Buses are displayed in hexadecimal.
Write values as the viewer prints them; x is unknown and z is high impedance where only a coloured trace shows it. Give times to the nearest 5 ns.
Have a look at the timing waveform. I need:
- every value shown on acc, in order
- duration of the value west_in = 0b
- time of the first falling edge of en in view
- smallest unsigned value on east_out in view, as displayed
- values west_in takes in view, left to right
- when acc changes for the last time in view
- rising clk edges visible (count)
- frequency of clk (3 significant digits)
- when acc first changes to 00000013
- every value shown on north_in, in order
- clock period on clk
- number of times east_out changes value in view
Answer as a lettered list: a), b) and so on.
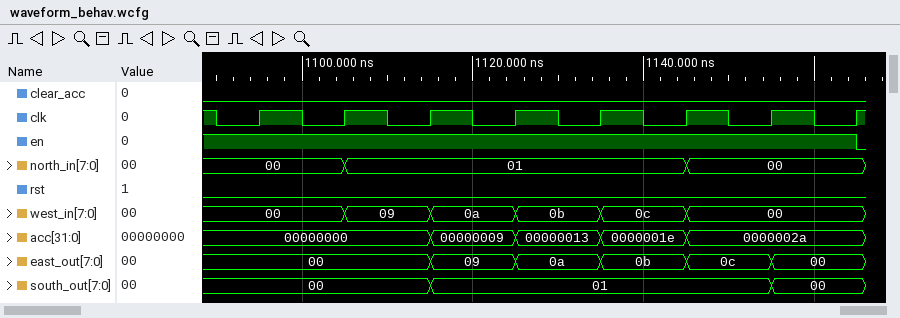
a) 00000000, 00000009, 00000013, 0000001e, 0000002a
b) 10 ns
c) 1165 ns
d) 00
e) 00, 09, 0a, 0b, 0c, 00
f) 1145 ns
g) 8
h) 100 MHz
i) 1125 ns
j) 00, 01, 00
k) 10 ns
l) 5
